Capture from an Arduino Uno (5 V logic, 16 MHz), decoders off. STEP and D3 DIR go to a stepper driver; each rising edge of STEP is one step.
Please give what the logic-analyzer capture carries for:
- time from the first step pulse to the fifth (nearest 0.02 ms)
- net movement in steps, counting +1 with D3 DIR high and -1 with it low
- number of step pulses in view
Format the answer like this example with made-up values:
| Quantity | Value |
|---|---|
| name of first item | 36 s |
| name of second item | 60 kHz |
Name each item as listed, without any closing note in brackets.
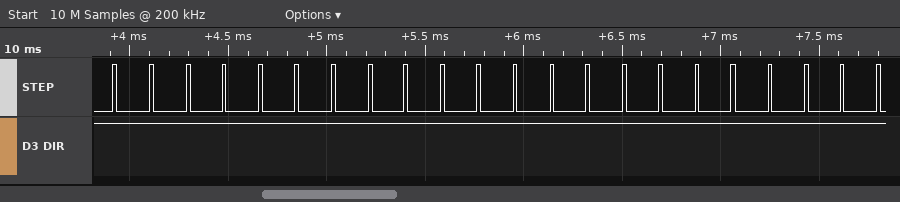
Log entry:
| Quantity | Value |
|---|---|
| time from the first step pulse to the fifth | 0.74 ms |
| net movement in steps, counting +1 with D3 DIR high and -1 with it low | +22 |
| number of step pulses in view | 22 |
